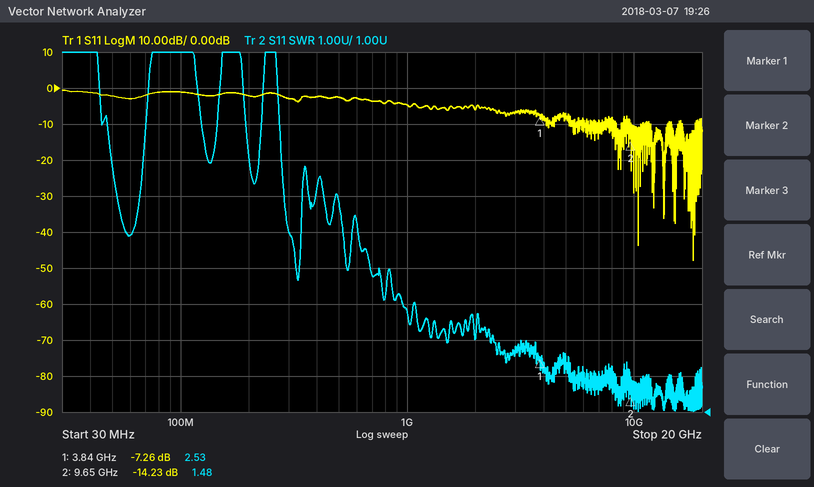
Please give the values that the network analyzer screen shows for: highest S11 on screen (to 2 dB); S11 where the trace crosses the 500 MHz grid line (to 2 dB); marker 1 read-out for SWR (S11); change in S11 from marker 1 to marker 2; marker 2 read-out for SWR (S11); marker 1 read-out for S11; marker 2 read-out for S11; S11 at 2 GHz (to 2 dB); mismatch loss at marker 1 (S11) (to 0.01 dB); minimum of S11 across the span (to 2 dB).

0 dB
-2 dB
2.53
-6.97 dB
1.48
-7.26 dB
-14.23 dB
-6 dB
0.90 dB
-48 dB
